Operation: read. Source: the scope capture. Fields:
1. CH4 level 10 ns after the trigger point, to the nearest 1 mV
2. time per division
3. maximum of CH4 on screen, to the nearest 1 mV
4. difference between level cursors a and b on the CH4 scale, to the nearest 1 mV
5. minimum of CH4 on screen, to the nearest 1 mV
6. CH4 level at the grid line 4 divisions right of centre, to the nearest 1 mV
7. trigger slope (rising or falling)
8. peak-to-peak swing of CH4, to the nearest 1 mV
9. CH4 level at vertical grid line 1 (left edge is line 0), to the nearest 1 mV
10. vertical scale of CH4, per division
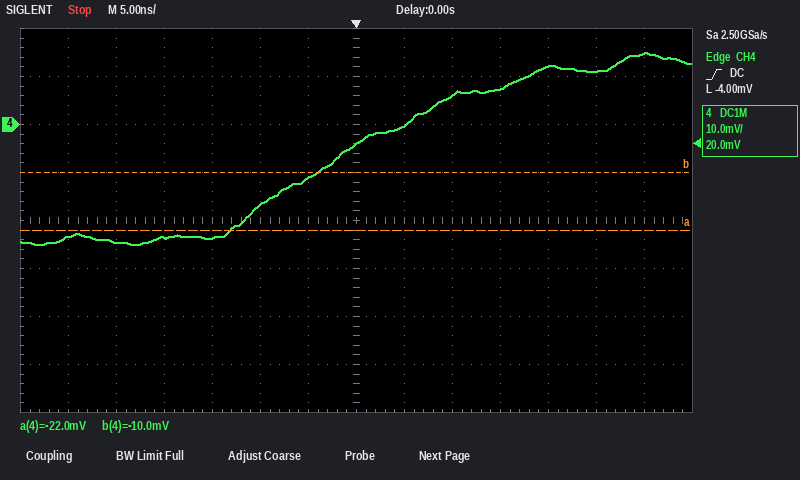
6 mV
5 ns
15 mV
12 mV
-25 mV
12 mV
rising
40 mV
-23 mV
10 mV
